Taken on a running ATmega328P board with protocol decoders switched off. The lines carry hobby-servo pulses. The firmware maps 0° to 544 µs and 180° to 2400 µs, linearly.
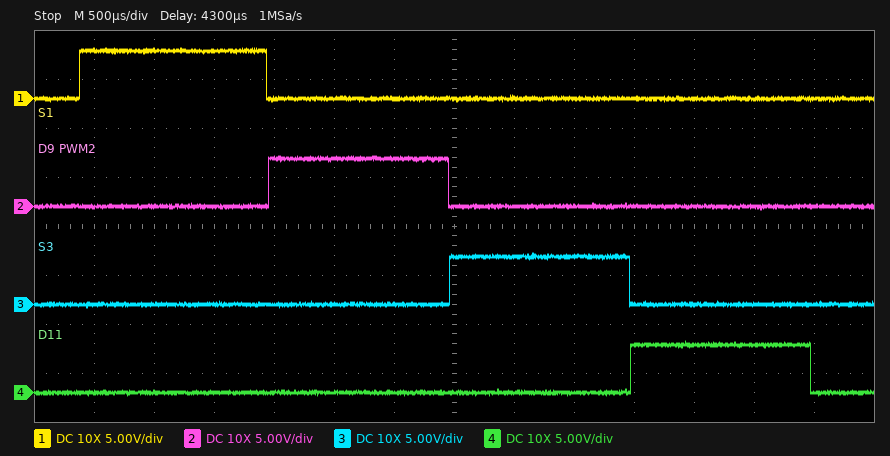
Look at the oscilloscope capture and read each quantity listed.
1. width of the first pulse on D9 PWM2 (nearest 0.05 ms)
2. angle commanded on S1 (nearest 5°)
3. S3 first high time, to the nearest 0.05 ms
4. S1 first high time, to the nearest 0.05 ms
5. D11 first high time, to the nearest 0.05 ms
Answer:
1.50 ms
100°
1.50 ms
1.55 ms
1.50 ms
